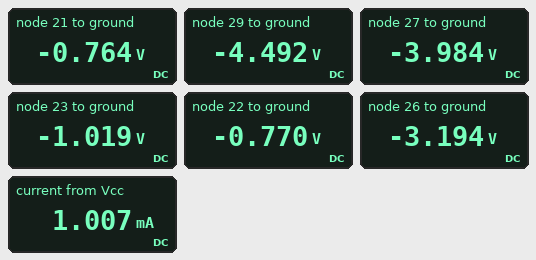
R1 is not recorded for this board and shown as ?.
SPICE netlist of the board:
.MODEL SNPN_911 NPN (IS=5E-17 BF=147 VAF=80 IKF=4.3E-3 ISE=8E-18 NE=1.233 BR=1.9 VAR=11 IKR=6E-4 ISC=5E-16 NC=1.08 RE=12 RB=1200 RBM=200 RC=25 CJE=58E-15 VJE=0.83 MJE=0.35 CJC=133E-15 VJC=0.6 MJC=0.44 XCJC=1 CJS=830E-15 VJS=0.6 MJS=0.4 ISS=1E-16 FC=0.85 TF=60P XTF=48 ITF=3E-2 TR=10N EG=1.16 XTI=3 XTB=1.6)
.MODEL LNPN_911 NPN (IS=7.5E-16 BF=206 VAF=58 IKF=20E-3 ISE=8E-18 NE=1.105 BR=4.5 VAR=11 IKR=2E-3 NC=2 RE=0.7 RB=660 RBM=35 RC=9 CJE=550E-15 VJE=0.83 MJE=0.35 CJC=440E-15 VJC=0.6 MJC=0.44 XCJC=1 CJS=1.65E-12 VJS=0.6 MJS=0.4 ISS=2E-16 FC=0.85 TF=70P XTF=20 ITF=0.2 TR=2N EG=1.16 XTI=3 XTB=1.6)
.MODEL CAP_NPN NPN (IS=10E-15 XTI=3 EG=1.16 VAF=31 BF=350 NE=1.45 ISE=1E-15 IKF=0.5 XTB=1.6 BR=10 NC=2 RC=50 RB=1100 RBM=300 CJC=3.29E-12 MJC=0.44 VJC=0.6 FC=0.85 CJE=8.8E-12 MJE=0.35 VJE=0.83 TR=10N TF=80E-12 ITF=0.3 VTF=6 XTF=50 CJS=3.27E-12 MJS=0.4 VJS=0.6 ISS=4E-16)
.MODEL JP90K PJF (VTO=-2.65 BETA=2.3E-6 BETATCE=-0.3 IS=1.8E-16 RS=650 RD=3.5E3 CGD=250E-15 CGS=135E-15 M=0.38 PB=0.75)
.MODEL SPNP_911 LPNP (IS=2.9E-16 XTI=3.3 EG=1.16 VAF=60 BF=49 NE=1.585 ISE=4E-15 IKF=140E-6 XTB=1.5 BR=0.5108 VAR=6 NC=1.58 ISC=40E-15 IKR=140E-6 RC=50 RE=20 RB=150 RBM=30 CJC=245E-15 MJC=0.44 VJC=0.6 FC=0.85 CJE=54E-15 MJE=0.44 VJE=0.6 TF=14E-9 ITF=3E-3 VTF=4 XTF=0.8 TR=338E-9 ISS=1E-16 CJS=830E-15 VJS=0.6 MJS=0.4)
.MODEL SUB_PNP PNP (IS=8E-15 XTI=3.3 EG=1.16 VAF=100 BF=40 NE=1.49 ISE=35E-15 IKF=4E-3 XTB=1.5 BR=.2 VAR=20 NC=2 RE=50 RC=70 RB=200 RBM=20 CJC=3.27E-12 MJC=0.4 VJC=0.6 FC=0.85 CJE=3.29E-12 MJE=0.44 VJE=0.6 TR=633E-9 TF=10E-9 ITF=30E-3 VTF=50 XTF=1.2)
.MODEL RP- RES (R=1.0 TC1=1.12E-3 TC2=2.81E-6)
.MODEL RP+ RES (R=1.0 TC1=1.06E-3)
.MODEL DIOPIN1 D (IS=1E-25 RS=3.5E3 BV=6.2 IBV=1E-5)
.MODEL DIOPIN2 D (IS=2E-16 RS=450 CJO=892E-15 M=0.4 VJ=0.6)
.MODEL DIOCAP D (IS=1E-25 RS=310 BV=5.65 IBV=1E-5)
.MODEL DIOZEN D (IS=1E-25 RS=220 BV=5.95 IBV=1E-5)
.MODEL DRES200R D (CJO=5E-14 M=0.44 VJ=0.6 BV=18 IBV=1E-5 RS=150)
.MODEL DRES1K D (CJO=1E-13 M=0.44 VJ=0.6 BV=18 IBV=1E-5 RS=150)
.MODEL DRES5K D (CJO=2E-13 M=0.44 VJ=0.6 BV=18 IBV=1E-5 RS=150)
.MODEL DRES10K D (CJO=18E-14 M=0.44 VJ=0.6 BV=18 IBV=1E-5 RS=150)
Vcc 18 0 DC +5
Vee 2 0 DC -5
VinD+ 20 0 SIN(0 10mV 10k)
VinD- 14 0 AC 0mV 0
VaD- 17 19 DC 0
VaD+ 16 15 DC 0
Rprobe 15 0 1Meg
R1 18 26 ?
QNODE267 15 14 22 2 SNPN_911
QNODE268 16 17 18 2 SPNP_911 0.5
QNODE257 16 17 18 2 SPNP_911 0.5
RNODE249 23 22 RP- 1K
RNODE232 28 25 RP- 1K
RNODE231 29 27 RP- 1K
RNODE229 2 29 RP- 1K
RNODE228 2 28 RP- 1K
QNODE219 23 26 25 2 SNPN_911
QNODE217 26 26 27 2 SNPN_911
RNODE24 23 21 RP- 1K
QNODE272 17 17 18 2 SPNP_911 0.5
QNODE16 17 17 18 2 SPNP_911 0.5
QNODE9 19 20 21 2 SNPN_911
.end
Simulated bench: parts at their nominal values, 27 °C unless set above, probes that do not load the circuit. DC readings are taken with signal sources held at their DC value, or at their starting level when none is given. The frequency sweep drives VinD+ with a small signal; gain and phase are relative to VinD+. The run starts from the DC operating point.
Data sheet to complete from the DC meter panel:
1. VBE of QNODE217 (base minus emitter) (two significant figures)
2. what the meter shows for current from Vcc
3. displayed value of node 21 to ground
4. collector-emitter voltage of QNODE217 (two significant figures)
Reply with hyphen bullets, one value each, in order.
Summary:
- 790 mV
- 1.007 mA
- -0.764 V
- 790 mV
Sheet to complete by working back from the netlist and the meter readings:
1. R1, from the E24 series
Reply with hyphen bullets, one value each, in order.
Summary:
- 16 kΩ
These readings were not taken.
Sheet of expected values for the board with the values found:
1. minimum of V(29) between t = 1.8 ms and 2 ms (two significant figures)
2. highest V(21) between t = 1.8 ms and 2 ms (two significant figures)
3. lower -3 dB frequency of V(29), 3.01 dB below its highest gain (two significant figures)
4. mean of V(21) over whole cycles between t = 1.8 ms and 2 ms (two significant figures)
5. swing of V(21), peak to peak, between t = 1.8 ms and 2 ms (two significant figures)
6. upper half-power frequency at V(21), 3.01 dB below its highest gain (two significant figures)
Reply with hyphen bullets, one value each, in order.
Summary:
- -4.5 V
- -750 mV
- 88 MHz
- -760 mV
- 19 mV
- 1.0 GHz
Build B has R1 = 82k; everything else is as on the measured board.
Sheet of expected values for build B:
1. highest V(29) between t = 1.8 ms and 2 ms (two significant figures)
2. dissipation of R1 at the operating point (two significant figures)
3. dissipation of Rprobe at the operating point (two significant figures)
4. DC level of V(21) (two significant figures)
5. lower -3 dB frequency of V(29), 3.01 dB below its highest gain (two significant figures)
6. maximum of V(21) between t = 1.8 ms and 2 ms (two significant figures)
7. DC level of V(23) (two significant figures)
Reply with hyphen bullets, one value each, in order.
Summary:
- -4.9 V
- 1.0 mW
- 510 nW
- -720 mV
- 73 MHz
- -710 mV
- -770 mV
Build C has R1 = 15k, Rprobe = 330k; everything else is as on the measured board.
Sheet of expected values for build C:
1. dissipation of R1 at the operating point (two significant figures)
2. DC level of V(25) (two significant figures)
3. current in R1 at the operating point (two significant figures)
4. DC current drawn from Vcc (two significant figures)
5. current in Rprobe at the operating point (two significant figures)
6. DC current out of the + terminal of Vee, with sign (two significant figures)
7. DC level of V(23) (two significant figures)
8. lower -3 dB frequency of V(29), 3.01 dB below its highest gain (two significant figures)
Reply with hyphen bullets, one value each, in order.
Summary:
- 4.4 mW
- -3.9 V
- 540 µA
- 1.1 mA
- 1.9 µA
- -1.1 mA
- -1.0 V
- 89 MHz
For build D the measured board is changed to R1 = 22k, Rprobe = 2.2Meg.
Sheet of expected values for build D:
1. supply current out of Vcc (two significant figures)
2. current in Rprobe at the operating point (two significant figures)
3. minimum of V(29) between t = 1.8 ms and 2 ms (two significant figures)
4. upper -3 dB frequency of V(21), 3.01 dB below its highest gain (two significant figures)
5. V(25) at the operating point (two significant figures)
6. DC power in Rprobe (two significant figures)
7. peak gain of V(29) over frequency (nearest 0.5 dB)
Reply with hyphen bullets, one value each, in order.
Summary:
- 760 µA
- 270 nA
- -4.6 V
- 970 MHz
- -4.2 V
- 160 nW
- -33.0 dB
